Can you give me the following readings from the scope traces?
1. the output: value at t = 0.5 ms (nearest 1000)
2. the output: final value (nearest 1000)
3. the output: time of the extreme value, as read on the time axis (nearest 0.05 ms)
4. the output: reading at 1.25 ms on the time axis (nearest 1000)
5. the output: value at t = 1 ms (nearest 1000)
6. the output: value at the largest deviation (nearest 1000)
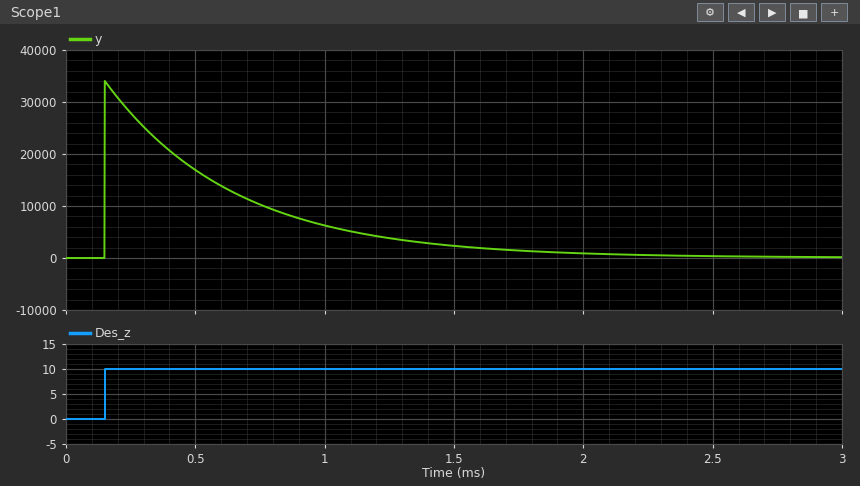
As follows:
17000
0
0.15 ms
4000
6000
34000
